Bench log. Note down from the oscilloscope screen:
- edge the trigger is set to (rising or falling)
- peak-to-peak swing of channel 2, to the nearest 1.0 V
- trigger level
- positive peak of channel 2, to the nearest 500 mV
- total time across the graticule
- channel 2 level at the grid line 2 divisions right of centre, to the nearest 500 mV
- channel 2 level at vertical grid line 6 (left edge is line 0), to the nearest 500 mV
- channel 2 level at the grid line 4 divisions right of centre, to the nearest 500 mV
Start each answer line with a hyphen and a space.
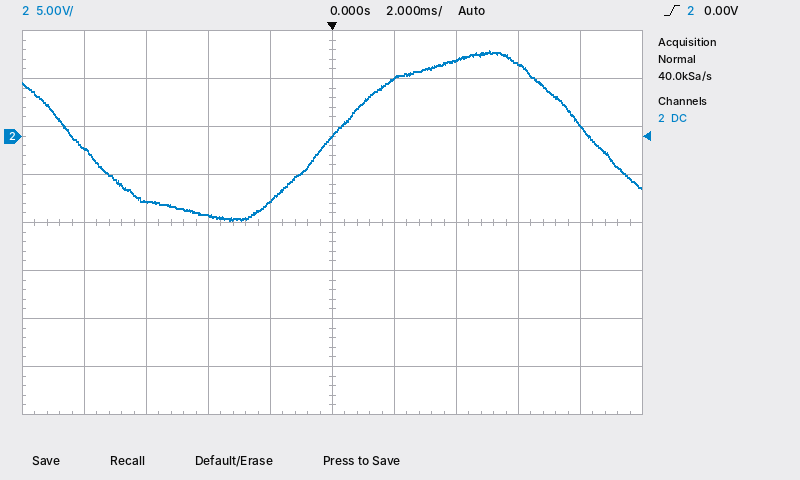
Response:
- rising
- 18.0 V
- 0.00 V
- 9.0 V
- 20 ms
- 8.0 V
- 6.0 V
- 1.0 V
